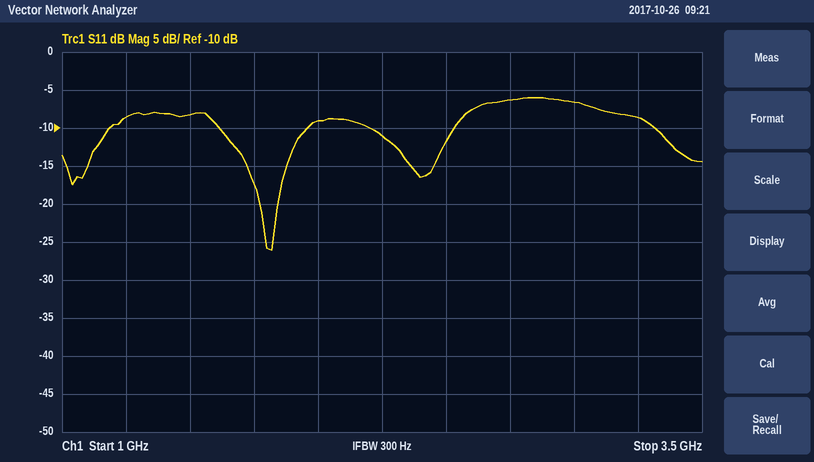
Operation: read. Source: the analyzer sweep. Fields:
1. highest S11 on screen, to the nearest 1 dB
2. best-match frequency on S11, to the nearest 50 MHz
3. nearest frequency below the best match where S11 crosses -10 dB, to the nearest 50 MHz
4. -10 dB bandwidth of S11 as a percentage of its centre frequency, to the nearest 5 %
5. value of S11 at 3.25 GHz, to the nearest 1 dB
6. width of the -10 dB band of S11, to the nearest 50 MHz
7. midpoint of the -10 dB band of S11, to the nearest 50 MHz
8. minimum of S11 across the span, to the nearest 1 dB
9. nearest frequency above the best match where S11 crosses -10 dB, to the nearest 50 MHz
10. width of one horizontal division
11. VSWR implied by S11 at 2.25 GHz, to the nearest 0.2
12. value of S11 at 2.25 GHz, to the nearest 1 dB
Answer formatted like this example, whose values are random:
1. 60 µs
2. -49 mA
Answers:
1. -6 dB
2. 1.80 GHz
3. 1.60 GHz
4. 20 %
5. -9 dB
6. 350 MHz
7. 1.80 GHz
8. -26 dB
9. 1.95 GHz
10. 250 MHz
11. 1.8
12. -11 dB
